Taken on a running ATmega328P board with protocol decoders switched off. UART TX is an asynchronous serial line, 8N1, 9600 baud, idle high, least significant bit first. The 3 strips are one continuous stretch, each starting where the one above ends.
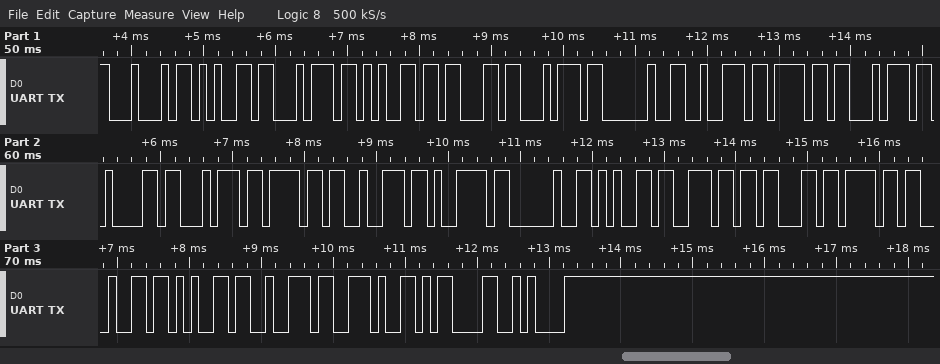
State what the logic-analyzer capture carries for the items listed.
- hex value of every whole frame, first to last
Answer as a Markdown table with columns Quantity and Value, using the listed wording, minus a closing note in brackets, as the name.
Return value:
| Quantity | Value |
|---|---|
| hex value of every whole frame, first to last | 44 65 74 65 63 74 20 72 6F 74 61 74 6F 72 79 20 65 6E 63 6F 64 65 72 2E 0D 0A |
